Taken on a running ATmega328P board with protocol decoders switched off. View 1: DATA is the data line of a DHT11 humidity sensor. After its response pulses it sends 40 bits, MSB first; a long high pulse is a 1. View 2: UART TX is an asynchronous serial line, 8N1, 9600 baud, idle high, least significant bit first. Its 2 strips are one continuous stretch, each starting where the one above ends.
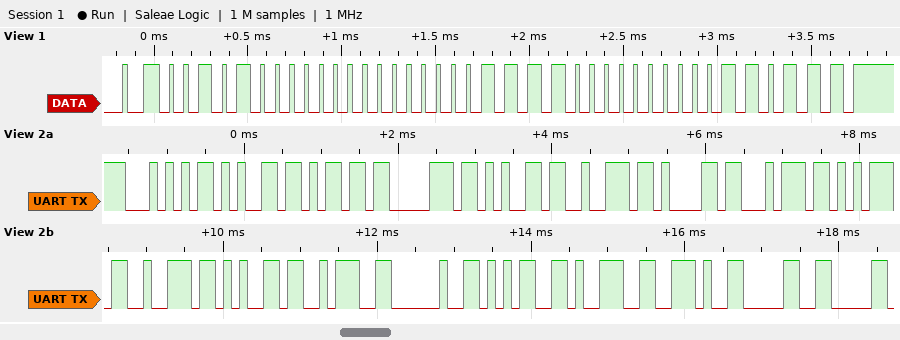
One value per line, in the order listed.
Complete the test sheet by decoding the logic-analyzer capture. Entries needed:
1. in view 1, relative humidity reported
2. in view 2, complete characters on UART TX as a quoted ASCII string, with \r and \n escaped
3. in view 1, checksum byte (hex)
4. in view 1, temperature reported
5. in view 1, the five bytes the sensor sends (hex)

40 %
"Temperature: 59.0"
0x37
15.0 °C
28 00 0F 00 37
